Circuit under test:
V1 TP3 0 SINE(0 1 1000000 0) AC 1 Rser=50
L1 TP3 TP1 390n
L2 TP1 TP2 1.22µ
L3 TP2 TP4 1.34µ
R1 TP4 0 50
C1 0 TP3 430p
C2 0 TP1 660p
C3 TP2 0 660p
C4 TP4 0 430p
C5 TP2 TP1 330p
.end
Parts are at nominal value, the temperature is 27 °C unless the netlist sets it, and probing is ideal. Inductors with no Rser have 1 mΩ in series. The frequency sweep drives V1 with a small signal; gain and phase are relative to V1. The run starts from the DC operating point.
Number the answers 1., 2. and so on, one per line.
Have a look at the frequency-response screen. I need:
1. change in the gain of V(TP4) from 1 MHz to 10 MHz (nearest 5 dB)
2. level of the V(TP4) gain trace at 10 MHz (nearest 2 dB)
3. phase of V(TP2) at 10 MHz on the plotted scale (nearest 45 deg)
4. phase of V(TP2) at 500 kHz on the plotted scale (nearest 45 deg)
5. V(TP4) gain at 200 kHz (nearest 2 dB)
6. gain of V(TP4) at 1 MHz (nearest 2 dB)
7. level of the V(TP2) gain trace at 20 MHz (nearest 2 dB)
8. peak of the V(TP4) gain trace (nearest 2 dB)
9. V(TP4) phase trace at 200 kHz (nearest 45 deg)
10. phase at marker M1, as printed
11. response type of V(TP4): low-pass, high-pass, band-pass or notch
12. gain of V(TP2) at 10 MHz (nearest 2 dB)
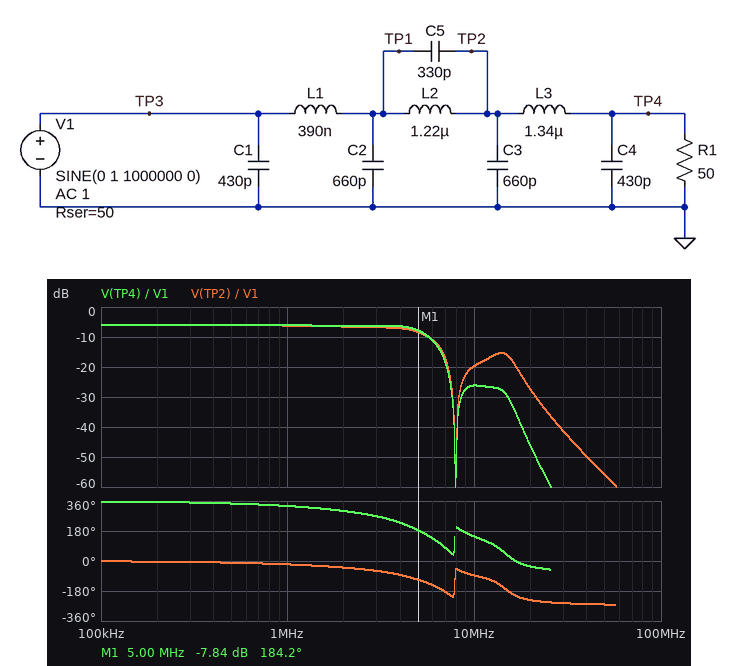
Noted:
1. -20 dB
2. -26 dB
3. -90 deg
4. 0 deg
5. -6 dB
6. -6 dB
7. -28 dB
8. -6 dB
9. 360 deg
10. 184.2 deg
11. low-pass
12. -20 dB
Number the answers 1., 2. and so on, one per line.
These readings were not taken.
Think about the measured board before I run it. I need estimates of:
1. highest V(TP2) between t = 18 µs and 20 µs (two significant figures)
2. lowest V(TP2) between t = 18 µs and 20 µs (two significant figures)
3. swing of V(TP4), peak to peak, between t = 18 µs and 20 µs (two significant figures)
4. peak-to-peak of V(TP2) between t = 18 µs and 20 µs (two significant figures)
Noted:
1. 490 mV
2. -490 mV
3. 990 mV
4. 980 mV
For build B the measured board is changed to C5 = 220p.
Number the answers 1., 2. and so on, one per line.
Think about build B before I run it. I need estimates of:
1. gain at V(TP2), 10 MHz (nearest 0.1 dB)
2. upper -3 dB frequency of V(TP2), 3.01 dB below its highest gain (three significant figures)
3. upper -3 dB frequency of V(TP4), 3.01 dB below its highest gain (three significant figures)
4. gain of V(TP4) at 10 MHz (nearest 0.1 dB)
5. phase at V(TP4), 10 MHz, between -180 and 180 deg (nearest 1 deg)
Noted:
1. -37.2 dB
2. 6.44 MHz
3. 6.08 MHz
4. -43.7 dB
5. 151 deg
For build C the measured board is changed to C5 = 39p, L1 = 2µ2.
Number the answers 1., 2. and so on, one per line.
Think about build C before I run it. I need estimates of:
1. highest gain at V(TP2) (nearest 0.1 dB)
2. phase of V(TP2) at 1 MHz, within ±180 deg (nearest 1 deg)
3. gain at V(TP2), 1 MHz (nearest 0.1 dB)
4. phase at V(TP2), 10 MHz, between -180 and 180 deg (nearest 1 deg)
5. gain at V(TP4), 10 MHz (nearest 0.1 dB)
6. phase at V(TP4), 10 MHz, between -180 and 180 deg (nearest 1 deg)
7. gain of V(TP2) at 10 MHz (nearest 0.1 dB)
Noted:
1. -4.2 dB
2. -27 deg
3. -6.1 dB
4. -17 deg
5. -20.1 dB
6. -144 deg
7. -13.6 dB
